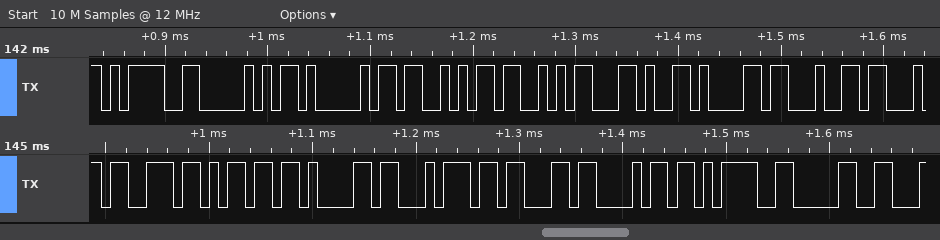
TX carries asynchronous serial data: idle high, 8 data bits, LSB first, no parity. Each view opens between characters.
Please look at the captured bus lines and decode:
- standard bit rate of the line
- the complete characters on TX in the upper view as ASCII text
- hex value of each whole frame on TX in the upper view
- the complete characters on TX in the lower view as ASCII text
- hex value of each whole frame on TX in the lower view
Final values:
115200 baud
"=PASS,ad"
3D, 50, 41, 53, 53, 2C, 61, 64
"smatch=0"
73, 6D, 61, 74, 63, 68, 3D, 30
